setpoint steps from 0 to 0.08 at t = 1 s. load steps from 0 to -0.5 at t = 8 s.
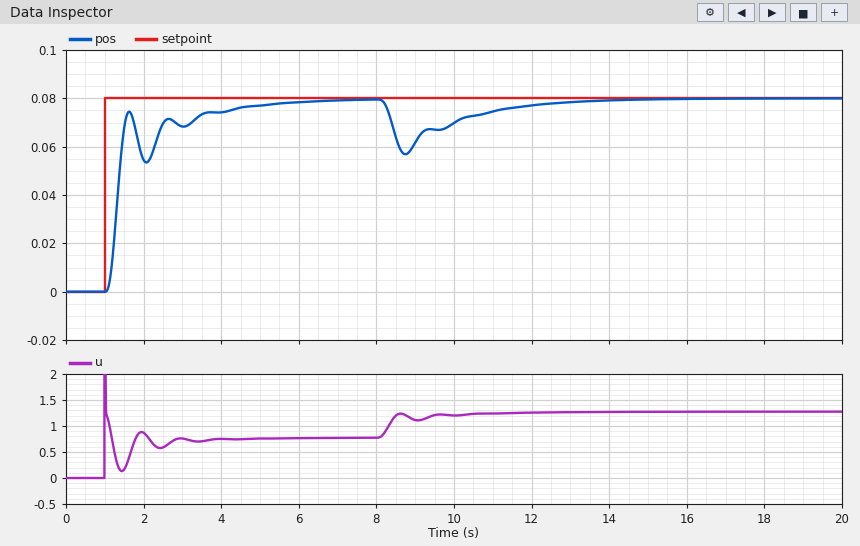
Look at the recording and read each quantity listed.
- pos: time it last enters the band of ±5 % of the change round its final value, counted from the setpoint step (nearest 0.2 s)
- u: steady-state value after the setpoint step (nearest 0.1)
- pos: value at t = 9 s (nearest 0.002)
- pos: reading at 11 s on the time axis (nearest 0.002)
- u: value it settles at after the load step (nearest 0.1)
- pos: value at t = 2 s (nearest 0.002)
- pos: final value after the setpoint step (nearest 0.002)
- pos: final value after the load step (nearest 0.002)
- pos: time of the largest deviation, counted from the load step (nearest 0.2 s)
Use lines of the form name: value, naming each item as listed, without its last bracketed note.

pos: time it last enters the band of ±5 % of the change round its final value, counted from the setpoint step: 3.4 s
u: steady-state value after the setpoint step: 0.8
pos: value at t = 9 s: 0.062
pos: reading at 11 s on the time axis: 0.074
u: value it settles at after the load step: 1.3
pos: value at t = 2 s: 0.054
pos: final value after the setpoint step: 0.080
pos: final value after the load step: 0.080
pos: time of the largest deviation, counted from the load step: 0.8 s
